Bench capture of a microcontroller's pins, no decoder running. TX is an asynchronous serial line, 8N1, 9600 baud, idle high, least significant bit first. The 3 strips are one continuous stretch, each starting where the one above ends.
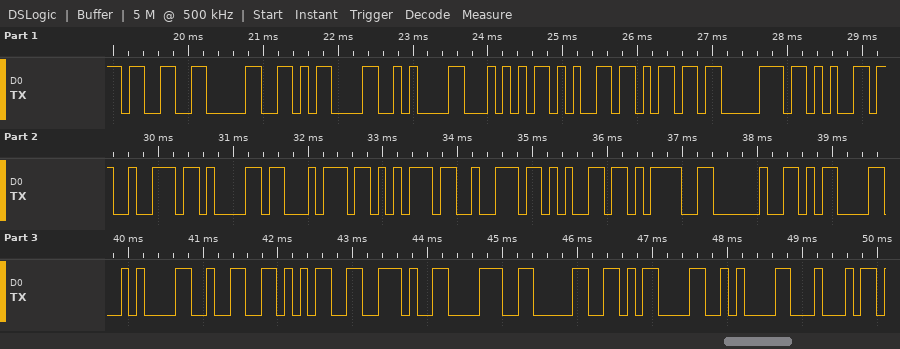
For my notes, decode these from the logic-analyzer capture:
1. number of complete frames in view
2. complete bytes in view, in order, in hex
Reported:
27
0x33 0x30 0x0D 0x0A 0x54 0x65 0x6D 0x70 0x65 0x72 0x61 0x74 0x75 0x72 0x65 0x3D 0x20 0x0D 0x0A 0x32 0x35 0x2E 0x38 0x30 0x0D 0x0A 0x44
